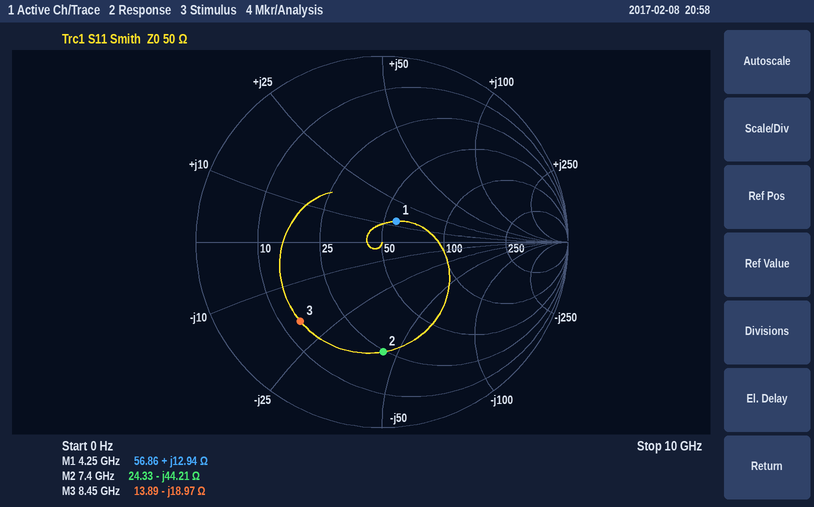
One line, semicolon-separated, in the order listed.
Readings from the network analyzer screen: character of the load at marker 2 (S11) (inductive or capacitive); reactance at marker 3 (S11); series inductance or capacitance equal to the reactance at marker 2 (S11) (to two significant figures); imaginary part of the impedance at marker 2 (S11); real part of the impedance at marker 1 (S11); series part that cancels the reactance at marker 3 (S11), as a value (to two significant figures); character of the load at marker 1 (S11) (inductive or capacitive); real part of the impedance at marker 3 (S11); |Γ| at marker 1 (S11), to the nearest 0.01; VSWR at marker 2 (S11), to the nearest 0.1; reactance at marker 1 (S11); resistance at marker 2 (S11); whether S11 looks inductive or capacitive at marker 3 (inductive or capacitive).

capacitive; -18.97 Ω; 490 fF; -44.21 Ω; 56.86 Ω; 360 pH; inductive; 13.89 Ω; 0.14; 3.9; +12.94 Ω; 24.33 Ω; capacitive
